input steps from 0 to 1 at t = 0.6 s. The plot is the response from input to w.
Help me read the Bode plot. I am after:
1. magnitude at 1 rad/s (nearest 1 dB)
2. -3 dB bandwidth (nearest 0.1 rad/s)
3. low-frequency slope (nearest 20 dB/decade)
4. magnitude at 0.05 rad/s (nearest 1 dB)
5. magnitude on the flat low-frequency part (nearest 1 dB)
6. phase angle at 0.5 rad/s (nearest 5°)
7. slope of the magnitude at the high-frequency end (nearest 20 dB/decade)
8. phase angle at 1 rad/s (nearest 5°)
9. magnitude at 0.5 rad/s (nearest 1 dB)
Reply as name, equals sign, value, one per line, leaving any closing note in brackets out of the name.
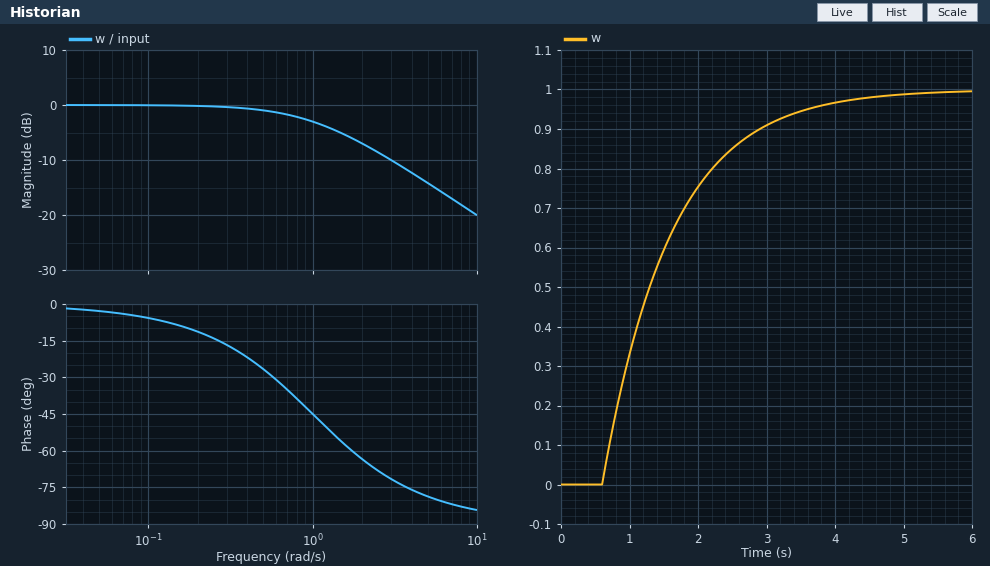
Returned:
magnitude at 1 rad/s = -3 dB
-3 dB bandwidth = 1.0 rad/s
low-frequency slope = 0 dB/decade
magnitude at 0.05 rad/s = 0 dB
magnitude on the flat low-frequency part = 0 dB
phase angle at 0.5 rad/s = -25°
slope of the magnitude at the high-frequency end = -20 dB/decade
phase angle at 1 rad/s = -45°
magnitude at 0.5 rad/s = -1 dB
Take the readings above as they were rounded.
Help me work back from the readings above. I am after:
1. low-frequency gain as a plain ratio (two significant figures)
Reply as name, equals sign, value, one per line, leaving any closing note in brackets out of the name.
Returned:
low-frequency gain as a plain ratio = 1.0
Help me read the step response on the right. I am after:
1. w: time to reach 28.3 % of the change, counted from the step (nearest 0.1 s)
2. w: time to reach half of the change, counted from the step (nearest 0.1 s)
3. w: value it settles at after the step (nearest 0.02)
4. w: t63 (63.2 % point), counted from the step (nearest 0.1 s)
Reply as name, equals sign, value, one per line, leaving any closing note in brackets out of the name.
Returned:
w: time to reach 28.3 % of the change, counted from the step = 0.3 s
w: time to reach half of the change, counted from the step = 0.7 s
w: value it settles at after the step = 1.00
w: t63 (63.2 % point), counted from the step = 1.0 s
